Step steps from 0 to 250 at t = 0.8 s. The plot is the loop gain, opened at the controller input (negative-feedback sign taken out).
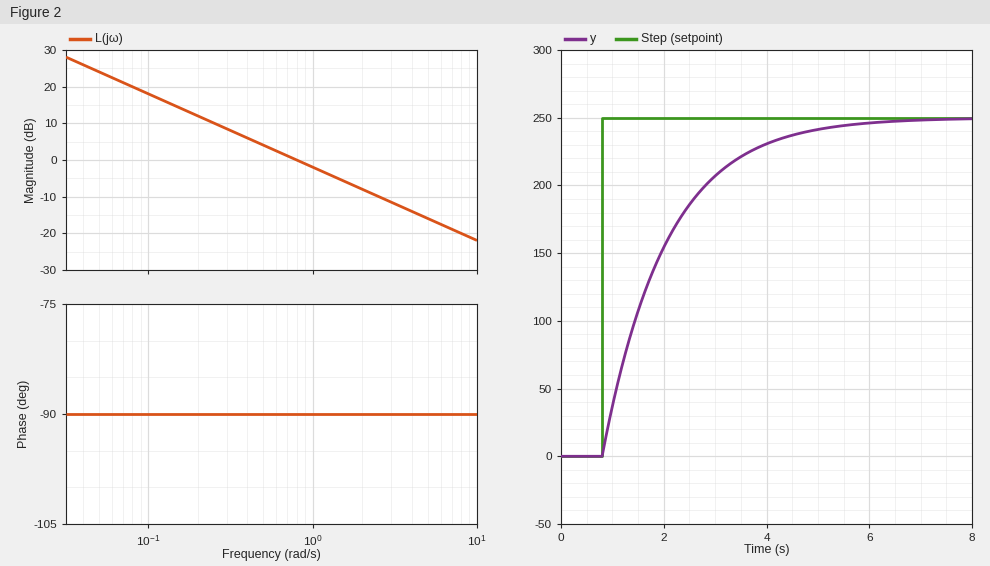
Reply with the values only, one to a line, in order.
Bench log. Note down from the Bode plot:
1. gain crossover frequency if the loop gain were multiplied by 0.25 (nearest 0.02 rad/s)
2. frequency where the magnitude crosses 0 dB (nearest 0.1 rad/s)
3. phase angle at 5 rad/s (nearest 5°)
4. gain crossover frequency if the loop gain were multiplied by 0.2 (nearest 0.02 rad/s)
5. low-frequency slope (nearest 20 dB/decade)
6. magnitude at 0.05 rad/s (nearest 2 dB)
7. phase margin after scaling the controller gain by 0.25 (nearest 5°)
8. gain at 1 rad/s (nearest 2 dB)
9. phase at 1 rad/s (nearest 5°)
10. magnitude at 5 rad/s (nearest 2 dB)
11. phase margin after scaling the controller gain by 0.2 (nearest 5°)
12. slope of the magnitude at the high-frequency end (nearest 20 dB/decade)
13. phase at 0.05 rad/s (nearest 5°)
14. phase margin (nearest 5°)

0.20 rad/s
0.8 rad/s
-90°
0.16 rad/s
-20 dB/decade
24 dB
90°
-2 dB
-90°
-16 dB
90°
-20 dB/decade
-90°
90°
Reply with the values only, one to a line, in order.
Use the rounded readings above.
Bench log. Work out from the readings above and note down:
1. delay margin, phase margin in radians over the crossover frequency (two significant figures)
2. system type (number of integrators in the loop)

2.0 s
1
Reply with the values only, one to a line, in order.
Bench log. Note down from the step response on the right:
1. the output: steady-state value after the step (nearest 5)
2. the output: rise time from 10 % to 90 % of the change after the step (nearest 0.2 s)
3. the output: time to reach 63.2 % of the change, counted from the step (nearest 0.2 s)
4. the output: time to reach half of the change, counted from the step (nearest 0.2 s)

250
2.8 s
1.2 s
0.8 s
